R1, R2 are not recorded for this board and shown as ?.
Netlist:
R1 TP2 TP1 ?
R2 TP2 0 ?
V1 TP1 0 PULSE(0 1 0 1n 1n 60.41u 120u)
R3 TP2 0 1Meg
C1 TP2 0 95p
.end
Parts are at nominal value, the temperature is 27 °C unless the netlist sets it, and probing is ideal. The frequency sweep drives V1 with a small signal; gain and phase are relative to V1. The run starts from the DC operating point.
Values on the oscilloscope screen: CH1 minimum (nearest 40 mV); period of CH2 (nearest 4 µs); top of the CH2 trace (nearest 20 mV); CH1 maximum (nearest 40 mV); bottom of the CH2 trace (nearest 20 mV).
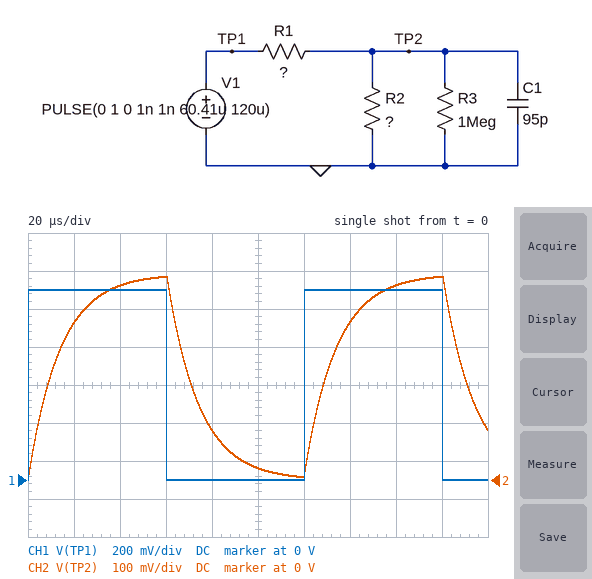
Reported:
0 V
120 µs
540 mV
1.00 V
0 V
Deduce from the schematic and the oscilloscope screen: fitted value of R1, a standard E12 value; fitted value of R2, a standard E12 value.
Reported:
270 kΩ
470 kΩ
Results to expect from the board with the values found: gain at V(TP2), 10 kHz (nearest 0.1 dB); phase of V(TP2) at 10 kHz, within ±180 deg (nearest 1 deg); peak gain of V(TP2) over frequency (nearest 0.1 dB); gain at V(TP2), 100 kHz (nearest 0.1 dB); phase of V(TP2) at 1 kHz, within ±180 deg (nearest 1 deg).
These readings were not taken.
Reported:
-7.8 dB
-41 deg
-5.3 dB
-24.2 dB
-5 deg
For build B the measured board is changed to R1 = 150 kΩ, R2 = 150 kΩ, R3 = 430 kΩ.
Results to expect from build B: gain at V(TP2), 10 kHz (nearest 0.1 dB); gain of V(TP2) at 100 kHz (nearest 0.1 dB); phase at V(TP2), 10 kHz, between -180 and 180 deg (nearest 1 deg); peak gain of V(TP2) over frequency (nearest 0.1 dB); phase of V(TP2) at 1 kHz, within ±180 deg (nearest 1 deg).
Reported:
-8.0 dB
-19.3 dB
-21 deg
-7.4 dB
-2 deg
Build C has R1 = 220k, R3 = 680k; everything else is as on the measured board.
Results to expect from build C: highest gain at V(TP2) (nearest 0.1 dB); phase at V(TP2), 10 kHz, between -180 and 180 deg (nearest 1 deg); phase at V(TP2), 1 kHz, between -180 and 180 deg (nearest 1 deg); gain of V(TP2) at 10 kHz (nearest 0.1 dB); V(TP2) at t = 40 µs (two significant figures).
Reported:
-5.1 dB
-36 deg
-4 deg
-6.9 dB
540 mV
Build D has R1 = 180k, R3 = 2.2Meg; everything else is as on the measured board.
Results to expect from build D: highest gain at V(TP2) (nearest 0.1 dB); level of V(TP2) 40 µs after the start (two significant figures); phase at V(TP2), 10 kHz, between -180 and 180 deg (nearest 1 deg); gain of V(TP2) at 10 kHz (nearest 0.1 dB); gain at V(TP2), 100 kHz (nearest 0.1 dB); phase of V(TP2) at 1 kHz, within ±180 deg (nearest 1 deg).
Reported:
-3.3 dB
660 mV
-36 deg
-5.2 dB
-20.7 dB
-4 deg
